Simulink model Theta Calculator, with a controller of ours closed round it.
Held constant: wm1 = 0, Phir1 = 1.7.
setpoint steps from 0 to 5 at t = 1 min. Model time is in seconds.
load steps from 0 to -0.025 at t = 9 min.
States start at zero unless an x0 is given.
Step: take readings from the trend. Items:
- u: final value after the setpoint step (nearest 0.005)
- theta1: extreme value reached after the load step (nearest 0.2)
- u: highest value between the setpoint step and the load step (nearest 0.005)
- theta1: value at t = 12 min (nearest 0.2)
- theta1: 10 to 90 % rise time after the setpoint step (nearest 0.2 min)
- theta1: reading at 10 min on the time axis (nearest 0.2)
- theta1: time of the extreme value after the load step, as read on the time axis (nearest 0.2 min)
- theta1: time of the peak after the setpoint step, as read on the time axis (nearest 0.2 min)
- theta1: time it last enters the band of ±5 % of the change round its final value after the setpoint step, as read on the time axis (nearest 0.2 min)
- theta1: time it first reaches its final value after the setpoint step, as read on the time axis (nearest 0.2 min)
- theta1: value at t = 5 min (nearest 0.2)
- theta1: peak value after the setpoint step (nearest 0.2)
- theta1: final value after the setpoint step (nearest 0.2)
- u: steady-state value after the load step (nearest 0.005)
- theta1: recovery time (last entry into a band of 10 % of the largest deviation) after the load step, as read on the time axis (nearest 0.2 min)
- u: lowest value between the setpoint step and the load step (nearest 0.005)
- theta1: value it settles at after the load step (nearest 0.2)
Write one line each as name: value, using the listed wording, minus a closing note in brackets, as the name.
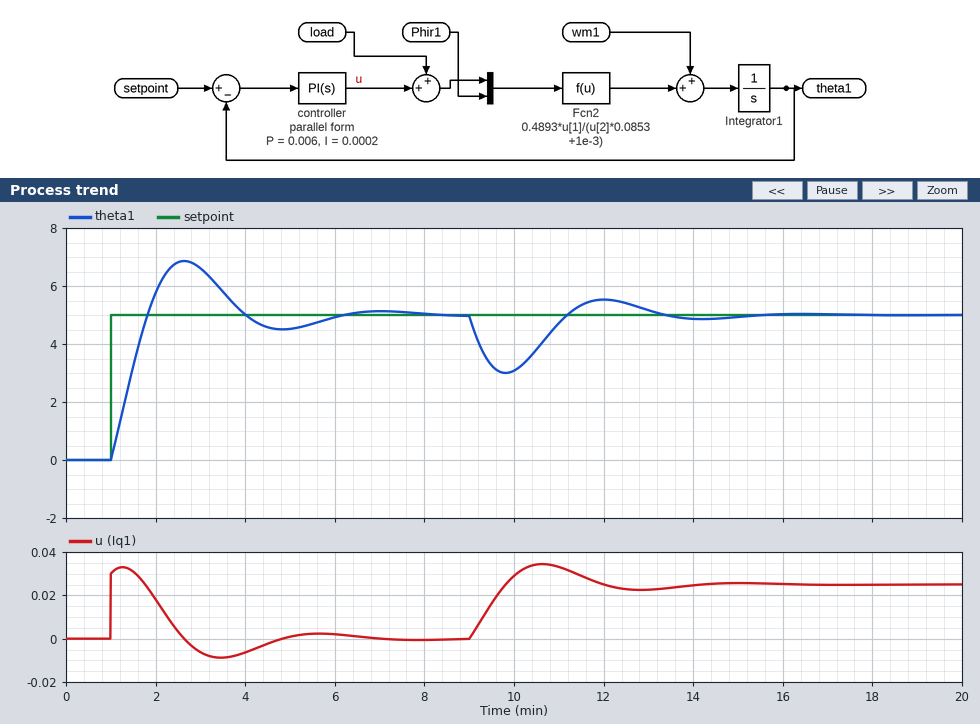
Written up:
u: final value after the setpoint step: 0.000
theta1: extreme value reached after the load step: 3.0
u: highest value between the setpoint step and the load step: 0.035
theta1: value at t = 12 min: 5.6
theta1: 10 to 90 % rise time after the setpoint step: 0.6 min
theta1: reading at 10 min on the time axis: 3.0
theta1: time of the extreme value after the load step, as read on the time axis: 9.8 min
theta1: time of the peak after the setpoint step, as read on the time axis: 2.6 min
theta1: time it last enters the band of ±5 % of the change round its final value after the setpoint step, as read on the time axis: 5.6 min
theta1: time it first reaches its final value after the setpoint step, as read on the time axis: 1.8 min
theta1: value at t = 5 min: 4.6
theta1: peak value after the setpoint step: 6.8
theta1: final value after the setpoint step: 5.0
u: steady-state value after the load step: 0.025
theta1: recovery time (last entry into a band of 10 % of the largest deviation) after the load step, as read on the time axis: 13.0 min
u: lowest value between the setpoint step and the load step: -0.010
theta1: value it settles at after the load step: 5.0
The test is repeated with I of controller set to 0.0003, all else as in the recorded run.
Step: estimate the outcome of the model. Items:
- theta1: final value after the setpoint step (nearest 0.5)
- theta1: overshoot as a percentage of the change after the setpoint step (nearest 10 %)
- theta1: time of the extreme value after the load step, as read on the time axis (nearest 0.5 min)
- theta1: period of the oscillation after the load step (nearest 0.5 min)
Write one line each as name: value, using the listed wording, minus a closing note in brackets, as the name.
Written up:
theta1: final value after the setpoint step: 5.0
theta1: overshoot as a percentage of the change after the setpoint step: 40 %
theta1: time of the extreme value after the load step, as read on the time axis: 9.5 min
theta1: period of the oscillation after the load step: 3.5 min
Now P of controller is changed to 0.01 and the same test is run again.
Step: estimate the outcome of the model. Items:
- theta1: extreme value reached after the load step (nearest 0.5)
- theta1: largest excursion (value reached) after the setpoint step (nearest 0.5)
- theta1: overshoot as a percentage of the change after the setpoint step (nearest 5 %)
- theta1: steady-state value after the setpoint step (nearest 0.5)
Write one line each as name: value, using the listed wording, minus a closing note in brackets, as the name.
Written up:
theta1: extreme value reached after the load step: 3.5
theta1: largest excursion (value reached) after the setpoint step: 6.0
theta1: overshoot as a percentage of the change after the setpoint step: 25 %
theta1: steady-state value after the setpoint step: 5.0
